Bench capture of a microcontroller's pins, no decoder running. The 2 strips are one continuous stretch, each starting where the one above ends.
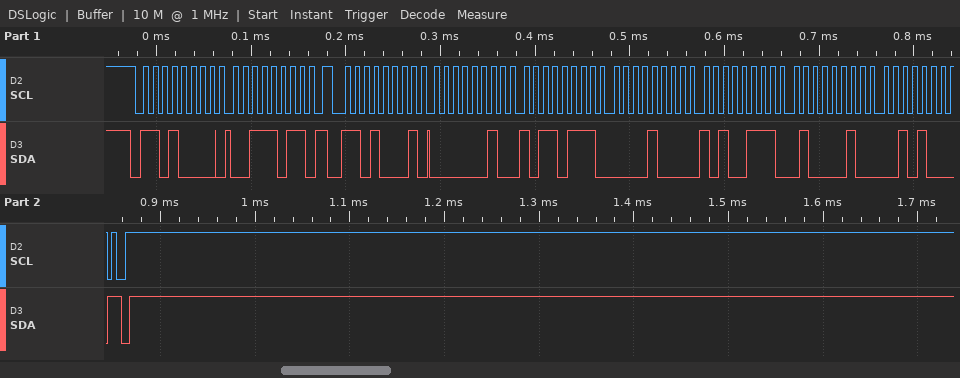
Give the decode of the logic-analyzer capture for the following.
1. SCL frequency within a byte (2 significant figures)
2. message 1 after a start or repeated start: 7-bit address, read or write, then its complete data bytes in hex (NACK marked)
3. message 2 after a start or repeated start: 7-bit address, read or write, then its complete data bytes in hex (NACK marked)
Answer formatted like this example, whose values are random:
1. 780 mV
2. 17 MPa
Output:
1. 100 kHz
2. 0x68 write: 3B
3. 0x68 read: 02 B7 08 A7 42 28 NACK
